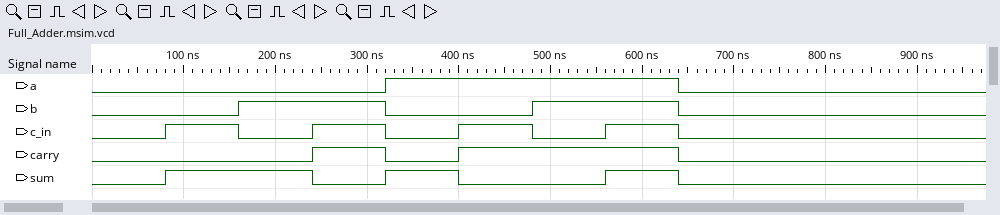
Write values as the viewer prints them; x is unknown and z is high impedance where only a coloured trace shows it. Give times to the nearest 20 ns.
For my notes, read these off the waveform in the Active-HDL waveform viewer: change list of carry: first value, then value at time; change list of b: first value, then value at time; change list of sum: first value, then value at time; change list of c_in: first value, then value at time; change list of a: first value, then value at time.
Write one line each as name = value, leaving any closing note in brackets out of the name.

change list of carry: first value, then value at time = 0, 1 at 240 ns, 0 at 320 ns, 1 at 400 ns, 0 at 640 ns
change list of b: first value, then value at time = 0, 1 at 160 ns, 0 at 320 ns, 1 at 480 ns, 0 at 640 ns
change list of sum: first value, then value at time = 0, 1 at 80 ns, 0 at 240 ns, 1 at 320 ns, 0 at 400 ns, 1 at 560 ns, 0 at 640 ns
change list of c_in: first value, then value at time = 0, 1 at 80 ns, 0 at 160 ns, 1 at 240 ns, 0 at 320 ns, 1 at 400 ns, 0 at 480 ns, 1 at 560 ns, 0 at 640 ns
change list of a: first value, then value at time = 0, 1 at 320 ns, 0 at 640 ns
